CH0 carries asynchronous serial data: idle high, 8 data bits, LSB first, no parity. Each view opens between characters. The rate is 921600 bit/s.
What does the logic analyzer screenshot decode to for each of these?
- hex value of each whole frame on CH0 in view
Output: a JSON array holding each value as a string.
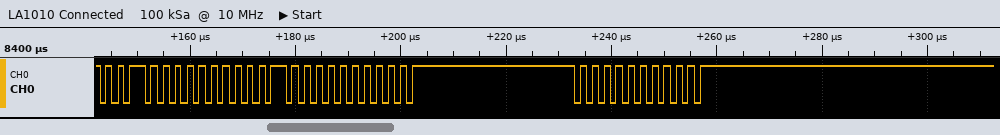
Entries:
["75, 55, 55, 55, 55, FF, 55, 55, FF"]
